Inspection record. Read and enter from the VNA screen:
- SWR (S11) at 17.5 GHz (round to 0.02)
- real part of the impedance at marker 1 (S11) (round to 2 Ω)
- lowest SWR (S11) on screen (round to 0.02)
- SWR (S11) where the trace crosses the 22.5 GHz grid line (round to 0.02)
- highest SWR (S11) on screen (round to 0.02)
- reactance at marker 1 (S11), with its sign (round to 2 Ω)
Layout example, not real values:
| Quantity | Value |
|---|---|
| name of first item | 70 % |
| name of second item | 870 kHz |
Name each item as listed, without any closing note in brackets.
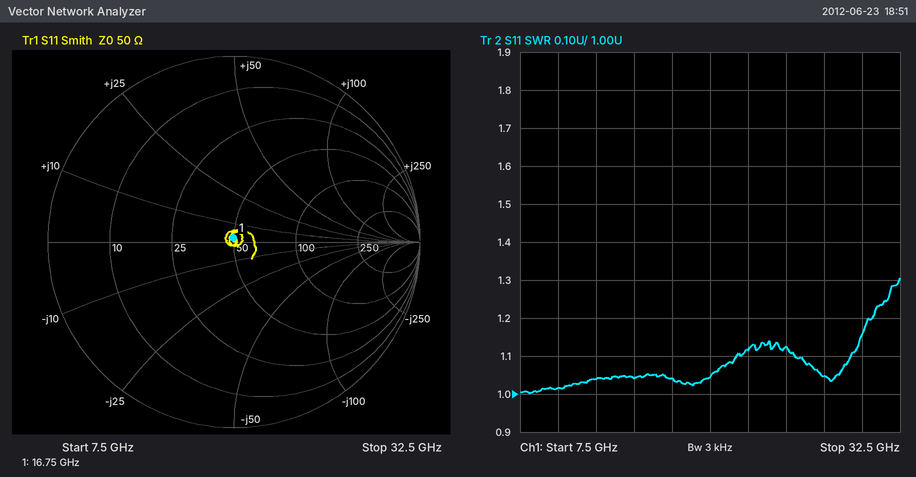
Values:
| Quantity | Value |
|---|---|
| SWR (S11) at 17.5 GHz | 1.04 |
| real part of the impedance at marker 1 (S11) | 50 Ω |
| lowest SWR (S11) on screen | 1.00 |
| SWR (S11) where the trace crosses the 22.5 GHz grid line | 1.12 |
| highest SWR (S11) on screen | 1.30 |
| reactance at marker 1 (S11), with its sign | +2 Ω |
